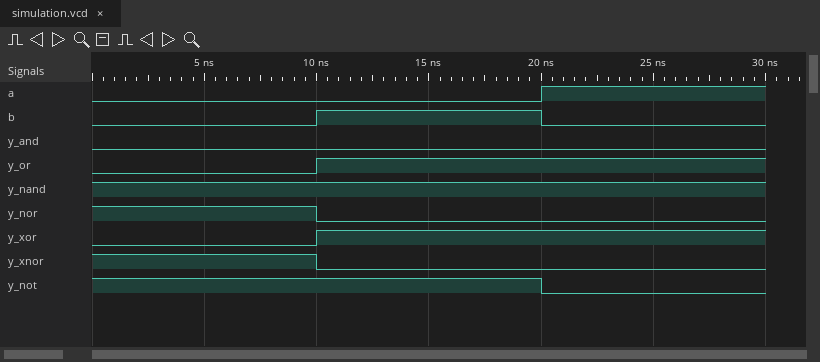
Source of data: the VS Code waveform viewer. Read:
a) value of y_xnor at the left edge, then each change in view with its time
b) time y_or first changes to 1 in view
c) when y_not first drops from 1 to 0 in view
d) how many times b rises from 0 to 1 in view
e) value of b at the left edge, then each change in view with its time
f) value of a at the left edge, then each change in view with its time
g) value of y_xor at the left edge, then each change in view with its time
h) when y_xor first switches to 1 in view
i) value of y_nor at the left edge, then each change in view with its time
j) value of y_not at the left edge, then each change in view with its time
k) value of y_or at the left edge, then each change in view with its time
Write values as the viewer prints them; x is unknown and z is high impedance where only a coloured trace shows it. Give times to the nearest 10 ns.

1, 0 at 10 ns
10 ns
20 ns
1
0, 1 at 10 ns, 0 at 20 ns
0, 1 at 20 ns
0, 1 at 10 ns
10 ns
1, 0 at 10 ns
1, 0 at 20 ns
0, 1 at 10 ns
